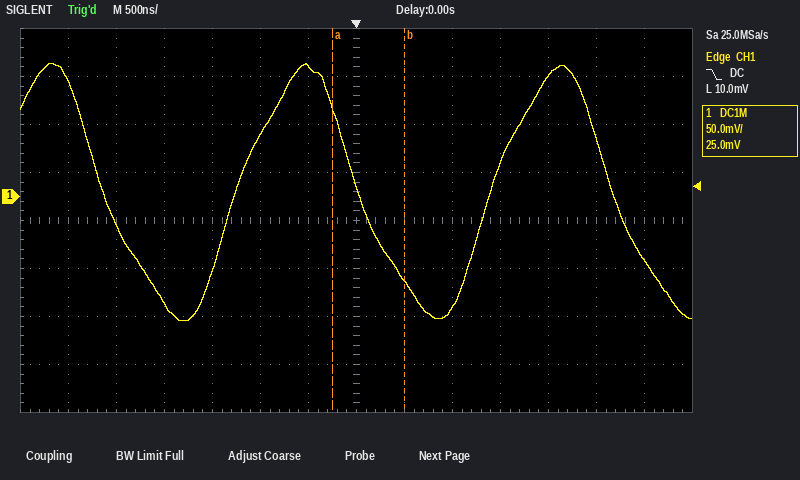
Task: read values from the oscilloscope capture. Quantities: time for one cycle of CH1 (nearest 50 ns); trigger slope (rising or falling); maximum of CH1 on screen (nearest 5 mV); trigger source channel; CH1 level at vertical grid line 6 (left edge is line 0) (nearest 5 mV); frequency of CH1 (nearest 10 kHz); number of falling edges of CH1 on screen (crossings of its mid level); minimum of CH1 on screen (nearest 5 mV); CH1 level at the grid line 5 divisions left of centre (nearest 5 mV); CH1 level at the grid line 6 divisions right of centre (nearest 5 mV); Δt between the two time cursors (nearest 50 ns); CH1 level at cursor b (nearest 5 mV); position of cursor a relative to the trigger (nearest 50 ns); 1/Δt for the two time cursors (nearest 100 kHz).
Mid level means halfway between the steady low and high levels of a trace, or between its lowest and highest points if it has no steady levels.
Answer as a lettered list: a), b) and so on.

a) 2.65 µs
b) falling
c) 140 mV
d) CH1
e) 135 mV
f) 380 kHz
g) 3
h) -130 mV
i) -30 mV
j) -65 mV
k) 750 ns
l) -90 mV
m) -250 ns
n) 1.3 MHz
